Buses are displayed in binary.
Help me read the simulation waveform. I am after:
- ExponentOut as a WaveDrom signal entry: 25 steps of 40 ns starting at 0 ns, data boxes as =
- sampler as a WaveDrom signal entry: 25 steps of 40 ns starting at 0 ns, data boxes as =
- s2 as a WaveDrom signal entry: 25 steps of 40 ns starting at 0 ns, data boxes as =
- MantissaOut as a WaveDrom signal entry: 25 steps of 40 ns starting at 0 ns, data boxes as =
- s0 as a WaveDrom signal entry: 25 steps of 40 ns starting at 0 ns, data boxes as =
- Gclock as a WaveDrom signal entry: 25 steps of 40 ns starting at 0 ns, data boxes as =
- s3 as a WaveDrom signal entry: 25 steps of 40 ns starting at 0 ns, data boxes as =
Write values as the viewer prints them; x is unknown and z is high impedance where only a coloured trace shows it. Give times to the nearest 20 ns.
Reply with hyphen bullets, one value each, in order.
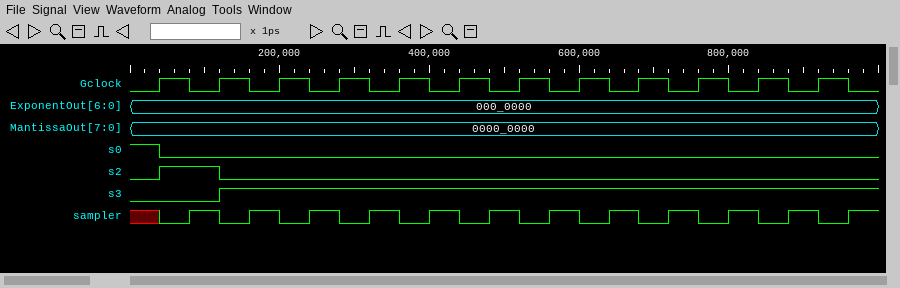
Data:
- {name: 'ExponentOut', wave: '=........................', data: '000_0000'}
- {name: 'sampler', wave: 'x010101010101010101010101'}
- {name: 's2', wave: '01.0.....................'}
- {name: 'MantissaOut', wave: '=........................', data: '0000_0000'}
- {name: 's0', wave: '10.......................'}
- {name: 'Gclock', wave: '0101010101010101010101010'}
- {name: 's3', wave: '0..1.....................'}
